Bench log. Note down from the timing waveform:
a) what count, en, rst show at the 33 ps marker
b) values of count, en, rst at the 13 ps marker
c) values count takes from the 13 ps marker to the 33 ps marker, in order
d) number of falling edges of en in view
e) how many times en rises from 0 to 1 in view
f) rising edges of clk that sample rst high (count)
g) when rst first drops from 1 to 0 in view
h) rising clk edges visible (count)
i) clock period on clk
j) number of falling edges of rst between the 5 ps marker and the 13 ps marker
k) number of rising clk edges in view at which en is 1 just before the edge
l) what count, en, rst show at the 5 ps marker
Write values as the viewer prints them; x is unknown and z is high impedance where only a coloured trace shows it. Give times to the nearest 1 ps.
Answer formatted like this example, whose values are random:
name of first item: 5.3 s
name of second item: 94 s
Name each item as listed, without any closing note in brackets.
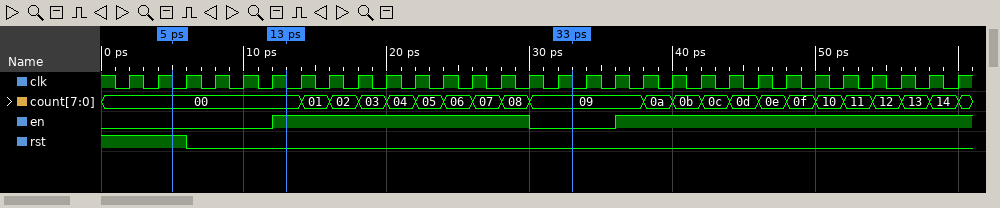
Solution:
what count, en, rst show at the 33 ps marker: count=09, en=0, rst=0
values of count, en, rst at the 13 ps marker: count=00, en=1, rst=0
values count takes from the 13 ps marker to the 33 ps marker, in order: 00, 01, 02, 03, 04, 05, 06, 07, 08, 09
number of falling edges of en in view: 1
how many times en rises from 0 to 1 in view: 2
rising edges of clk that sample rst high: 3
when rst first drops from 1 to 0 in view: 6 ps
rising clk edges visible: 30
clock period on clk: 2 ps
number of falling edges of rst between the 5 ps marker and the 13 ps marker: 1
number of rising clk edges in view at which en is 1 just before the edge: 21
what count, en, rst show at the 5 ps marker: count=00, en=0, rst=1
